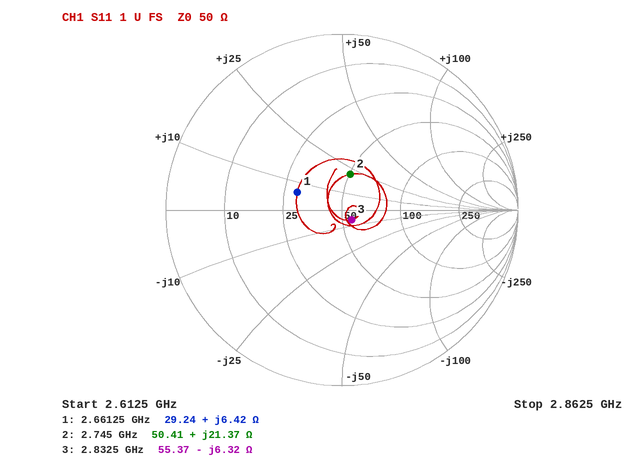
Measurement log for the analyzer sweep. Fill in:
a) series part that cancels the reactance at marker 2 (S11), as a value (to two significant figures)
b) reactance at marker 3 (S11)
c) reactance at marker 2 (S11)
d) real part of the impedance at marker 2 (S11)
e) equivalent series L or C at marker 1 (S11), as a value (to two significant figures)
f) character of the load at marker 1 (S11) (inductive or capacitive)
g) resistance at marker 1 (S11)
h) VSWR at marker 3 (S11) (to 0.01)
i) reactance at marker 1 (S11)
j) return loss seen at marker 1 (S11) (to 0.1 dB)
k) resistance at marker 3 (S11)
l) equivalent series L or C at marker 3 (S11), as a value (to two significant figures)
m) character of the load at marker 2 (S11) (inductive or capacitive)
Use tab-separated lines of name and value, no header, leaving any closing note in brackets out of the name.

series part that cancels the reactance at marker 2 (S11), as a value	2.7 pF
reactance at marker 3	-6.32 Ω
reactance at marker 2	+21.37 Ω
real part of the impedance at marker 2	50.41 Ω
equivalent series L or C at marker 1 (S11), as a value	380 pH
character of the load at marker 1 (S11)	inductive
resistance at marker 1	29.24 Ω
VSWR at marker 3 (S11)	1.17
reactance at marker 1	+6.42 Ω
return loss seen at marker 1 (S11)	11.3 dB
resistance at marker 3	55.37 Ω
equivalent series L or C at marker 3 (S11), as a value	8.9 pF
character of the load at marker 2 (S11)	inductive
